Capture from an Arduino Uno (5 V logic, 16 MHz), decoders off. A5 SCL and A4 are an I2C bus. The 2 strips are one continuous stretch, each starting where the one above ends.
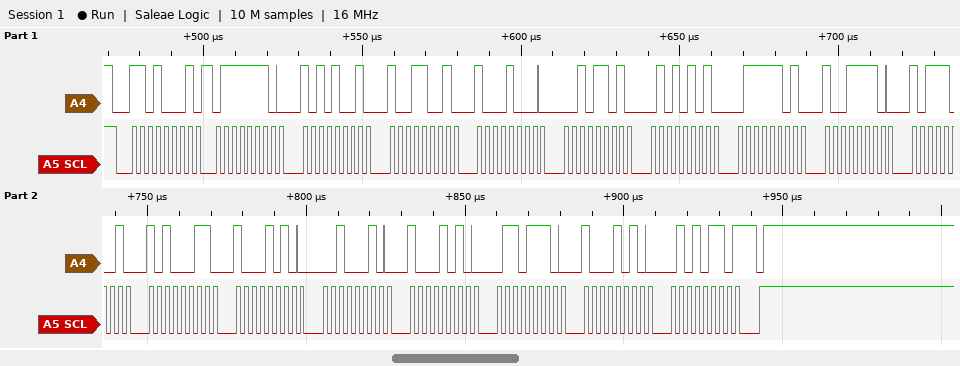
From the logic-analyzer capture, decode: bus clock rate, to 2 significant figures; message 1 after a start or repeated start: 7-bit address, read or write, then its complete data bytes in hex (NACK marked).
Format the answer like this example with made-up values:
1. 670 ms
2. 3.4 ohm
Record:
1. 400 kHz
2. 0x68 read: 7E A9 99 88 2D 55 7D 9E B9 A3 8A 22 8A 6E 8A 56 NACK
